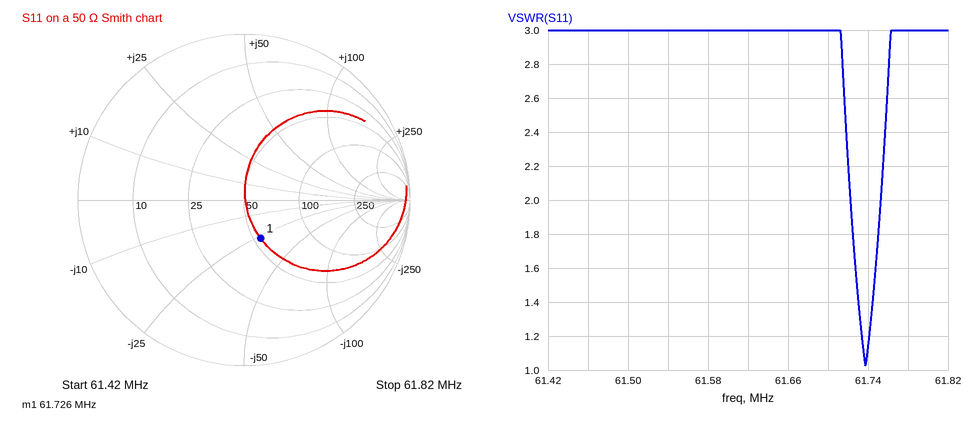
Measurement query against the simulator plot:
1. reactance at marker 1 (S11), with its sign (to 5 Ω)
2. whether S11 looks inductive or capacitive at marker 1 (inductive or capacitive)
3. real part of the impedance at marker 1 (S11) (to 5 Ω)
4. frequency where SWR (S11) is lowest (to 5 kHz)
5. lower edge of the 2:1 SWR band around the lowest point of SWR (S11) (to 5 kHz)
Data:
-25 Ω
capacitive
55 Ω
61.735 MHz
61.720 MHz
